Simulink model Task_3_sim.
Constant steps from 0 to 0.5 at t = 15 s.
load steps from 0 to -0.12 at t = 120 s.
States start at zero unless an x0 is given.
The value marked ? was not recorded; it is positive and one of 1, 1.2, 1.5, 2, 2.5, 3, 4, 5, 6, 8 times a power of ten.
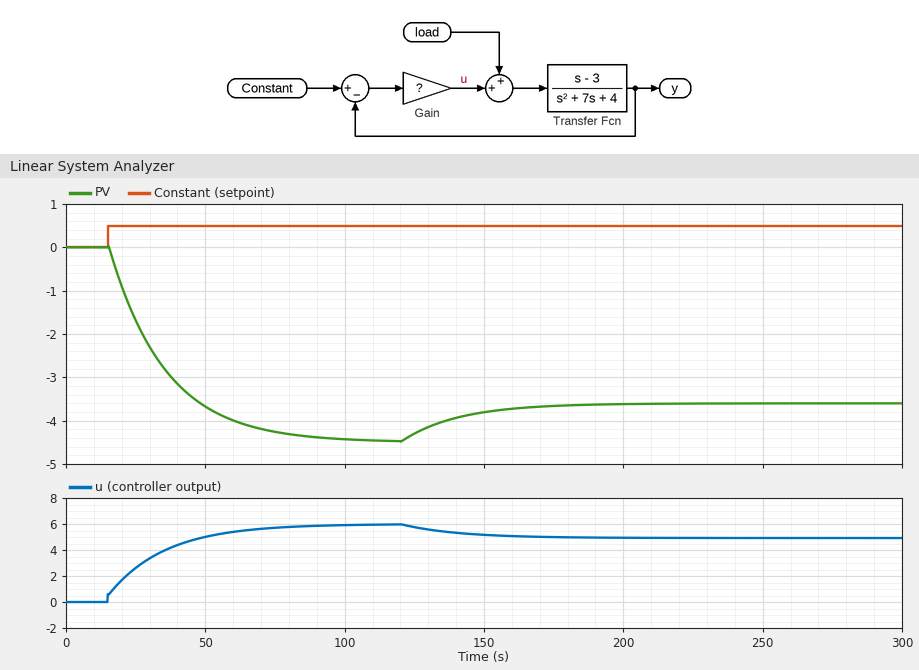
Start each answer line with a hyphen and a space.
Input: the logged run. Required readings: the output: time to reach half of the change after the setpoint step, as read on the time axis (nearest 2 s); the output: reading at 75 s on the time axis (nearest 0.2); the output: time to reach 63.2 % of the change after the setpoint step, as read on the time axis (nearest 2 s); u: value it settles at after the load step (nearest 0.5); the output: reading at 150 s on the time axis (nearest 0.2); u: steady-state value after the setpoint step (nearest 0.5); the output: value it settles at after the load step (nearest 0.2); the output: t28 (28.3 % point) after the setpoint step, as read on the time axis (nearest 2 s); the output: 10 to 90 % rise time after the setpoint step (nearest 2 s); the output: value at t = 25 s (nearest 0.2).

- 30 s
- -4.2
- 36 s
- 5.0
- -3.8
- 6.0
- -3.6
- 22 s
- 44 s
- -1.6
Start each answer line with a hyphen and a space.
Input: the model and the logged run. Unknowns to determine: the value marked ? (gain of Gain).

- 1.2
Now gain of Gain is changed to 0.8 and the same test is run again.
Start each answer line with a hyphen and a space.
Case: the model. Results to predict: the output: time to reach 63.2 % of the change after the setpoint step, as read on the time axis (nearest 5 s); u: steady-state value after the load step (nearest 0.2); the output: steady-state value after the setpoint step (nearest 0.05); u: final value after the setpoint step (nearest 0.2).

- 20 s
- 0.8
- -0.75
- 1.0
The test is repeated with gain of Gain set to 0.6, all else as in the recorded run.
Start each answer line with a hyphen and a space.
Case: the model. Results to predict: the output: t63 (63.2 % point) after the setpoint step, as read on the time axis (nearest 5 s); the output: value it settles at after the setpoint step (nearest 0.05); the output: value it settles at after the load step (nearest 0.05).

- 20 s
- -0.40
- -0.25
